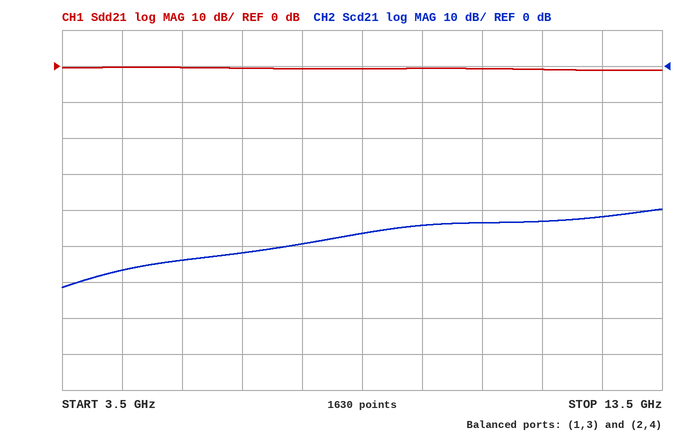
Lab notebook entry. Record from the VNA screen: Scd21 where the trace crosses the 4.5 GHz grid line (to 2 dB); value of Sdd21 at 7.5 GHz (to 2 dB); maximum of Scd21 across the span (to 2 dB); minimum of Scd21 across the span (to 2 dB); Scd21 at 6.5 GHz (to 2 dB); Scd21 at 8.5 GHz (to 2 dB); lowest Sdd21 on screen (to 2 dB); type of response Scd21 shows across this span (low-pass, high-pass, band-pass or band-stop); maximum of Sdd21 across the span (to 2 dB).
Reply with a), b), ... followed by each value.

a) -56 dB
b) 0 dB
c) -40 dB
d) -62 dB
e) -52 dB
f) -46 dB
g) -2 dB
h) high-pass
i) 0 dB
